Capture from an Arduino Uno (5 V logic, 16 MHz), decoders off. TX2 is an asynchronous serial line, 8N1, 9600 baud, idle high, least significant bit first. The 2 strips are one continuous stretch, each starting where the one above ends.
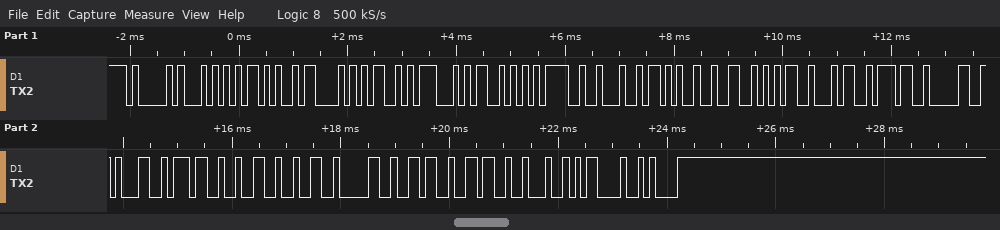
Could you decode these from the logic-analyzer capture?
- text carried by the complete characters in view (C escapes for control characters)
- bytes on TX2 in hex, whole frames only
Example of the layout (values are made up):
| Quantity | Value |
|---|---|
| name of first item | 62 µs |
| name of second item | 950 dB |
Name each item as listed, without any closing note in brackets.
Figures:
| Quantity | Value |
|---|---|
| text carried by the complete characters in view | "AT+CMGS=\"+254701722066\"\r\n" |
| bytes on TX2 in hex, whole frames only | 41 54 2B 43 4D 47 53 3D 22 2B 32 35 34 37 30 31 37 32 32 30 36 36 22 0D 0A |
